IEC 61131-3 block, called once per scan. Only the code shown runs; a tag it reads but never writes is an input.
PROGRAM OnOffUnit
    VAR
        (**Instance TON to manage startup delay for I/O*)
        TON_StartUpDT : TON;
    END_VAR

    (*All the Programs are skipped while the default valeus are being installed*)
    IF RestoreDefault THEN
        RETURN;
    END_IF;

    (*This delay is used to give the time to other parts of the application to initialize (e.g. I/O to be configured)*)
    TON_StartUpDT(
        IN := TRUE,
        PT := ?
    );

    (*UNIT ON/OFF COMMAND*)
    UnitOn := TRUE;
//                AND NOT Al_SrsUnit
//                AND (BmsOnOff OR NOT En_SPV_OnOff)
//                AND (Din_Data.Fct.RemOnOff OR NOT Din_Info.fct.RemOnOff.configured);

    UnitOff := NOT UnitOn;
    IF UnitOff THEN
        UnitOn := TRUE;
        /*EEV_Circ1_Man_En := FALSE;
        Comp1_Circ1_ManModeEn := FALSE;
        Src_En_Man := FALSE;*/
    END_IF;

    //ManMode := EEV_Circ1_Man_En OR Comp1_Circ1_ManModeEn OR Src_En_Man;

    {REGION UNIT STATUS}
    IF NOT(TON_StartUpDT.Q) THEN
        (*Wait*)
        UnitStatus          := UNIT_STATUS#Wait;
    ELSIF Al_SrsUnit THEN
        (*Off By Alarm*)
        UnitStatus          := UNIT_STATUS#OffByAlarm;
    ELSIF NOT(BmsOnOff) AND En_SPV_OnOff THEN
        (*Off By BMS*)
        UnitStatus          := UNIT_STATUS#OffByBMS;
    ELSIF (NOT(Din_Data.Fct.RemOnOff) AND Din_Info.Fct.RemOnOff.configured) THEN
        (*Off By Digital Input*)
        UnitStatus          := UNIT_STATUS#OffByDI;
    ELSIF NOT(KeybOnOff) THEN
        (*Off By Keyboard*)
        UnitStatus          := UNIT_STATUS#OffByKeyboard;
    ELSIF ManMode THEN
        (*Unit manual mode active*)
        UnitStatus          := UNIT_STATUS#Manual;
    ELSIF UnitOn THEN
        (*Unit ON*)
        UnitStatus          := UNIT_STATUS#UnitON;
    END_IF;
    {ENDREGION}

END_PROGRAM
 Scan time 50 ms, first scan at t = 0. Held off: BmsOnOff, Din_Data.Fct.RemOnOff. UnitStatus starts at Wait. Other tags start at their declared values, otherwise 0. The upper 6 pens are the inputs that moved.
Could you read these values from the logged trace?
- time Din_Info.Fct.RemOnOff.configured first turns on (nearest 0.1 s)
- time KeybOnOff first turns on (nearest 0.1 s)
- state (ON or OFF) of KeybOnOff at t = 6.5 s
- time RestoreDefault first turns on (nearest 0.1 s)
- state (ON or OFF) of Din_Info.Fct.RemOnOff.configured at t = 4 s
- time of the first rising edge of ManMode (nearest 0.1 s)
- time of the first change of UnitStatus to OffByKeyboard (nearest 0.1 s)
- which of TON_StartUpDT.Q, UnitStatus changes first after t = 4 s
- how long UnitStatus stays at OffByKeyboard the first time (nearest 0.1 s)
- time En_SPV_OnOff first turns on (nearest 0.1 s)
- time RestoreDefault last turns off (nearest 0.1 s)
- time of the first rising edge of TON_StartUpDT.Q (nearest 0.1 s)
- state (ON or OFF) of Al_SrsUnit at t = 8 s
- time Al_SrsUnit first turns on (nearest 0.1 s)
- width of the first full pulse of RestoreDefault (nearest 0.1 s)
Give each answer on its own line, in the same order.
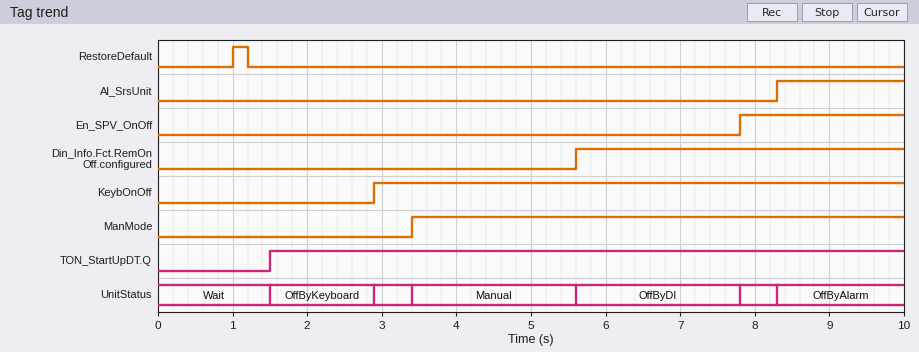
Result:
5.6 s
2.9 s
ON
1.0 s
OFF
3.4 s
1.5 s
UnitStatus
1.4 s
7.8 s
1.2 s
1.5 s
OFF
8.3 s
0.2 s
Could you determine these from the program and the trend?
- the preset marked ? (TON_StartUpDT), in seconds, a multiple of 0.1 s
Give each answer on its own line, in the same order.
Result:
1.5 s
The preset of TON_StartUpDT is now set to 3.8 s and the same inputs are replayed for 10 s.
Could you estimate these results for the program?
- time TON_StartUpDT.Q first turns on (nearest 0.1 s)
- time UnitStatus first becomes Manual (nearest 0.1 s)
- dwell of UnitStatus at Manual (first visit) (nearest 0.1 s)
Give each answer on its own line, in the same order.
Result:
3.8 s
3.8 s
1.8 s
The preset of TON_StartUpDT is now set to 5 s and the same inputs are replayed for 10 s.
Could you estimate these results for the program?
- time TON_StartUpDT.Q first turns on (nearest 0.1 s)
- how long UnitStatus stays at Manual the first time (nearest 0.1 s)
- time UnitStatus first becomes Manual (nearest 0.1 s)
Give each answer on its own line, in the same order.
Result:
5.0 s
0.6 s
5.0 s
